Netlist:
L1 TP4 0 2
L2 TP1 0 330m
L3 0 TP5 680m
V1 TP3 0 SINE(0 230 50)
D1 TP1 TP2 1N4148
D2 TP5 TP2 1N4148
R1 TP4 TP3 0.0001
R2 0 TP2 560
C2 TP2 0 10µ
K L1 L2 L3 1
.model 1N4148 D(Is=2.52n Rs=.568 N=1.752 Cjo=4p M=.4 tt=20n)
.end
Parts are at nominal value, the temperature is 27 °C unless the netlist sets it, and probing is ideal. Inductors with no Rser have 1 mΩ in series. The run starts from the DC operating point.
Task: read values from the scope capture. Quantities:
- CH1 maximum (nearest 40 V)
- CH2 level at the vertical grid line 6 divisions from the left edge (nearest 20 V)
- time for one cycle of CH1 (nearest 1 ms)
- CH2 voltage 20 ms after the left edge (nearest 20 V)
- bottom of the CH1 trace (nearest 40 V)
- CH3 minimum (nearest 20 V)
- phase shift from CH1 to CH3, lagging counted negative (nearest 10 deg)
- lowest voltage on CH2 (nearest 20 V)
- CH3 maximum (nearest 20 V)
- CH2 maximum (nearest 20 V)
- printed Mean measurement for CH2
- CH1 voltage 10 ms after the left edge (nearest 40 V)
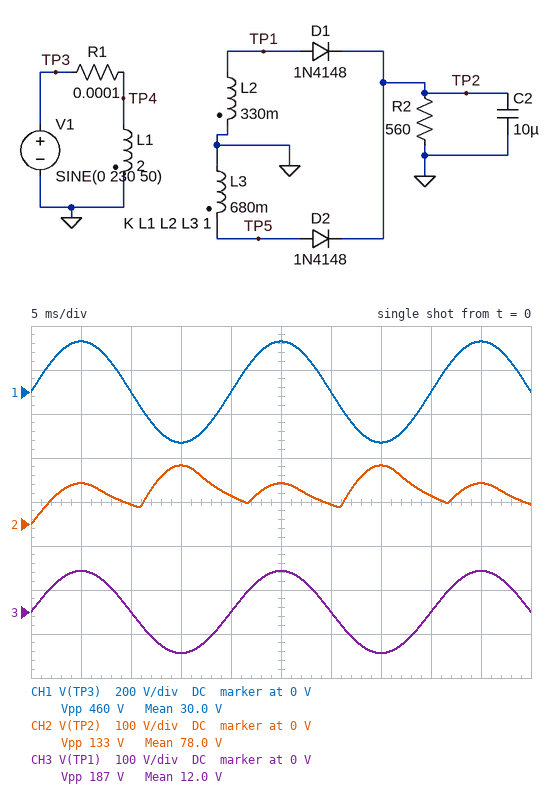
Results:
240 V
40 V
20 ms
60 V
-240 V
-100 V
0 deg
0 V
100 V
140 V
78.0 V
0 V
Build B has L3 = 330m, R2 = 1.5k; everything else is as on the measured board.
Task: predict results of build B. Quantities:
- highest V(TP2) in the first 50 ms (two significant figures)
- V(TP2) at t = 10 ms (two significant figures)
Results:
93 V
68 V
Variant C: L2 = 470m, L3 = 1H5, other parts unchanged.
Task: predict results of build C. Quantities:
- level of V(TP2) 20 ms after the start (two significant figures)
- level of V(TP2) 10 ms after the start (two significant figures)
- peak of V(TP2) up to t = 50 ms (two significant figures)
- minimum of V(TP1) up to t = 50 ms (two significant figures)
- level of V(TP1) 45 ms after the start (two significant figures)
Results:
95 V
53 V
200 V
-110 V
110 V
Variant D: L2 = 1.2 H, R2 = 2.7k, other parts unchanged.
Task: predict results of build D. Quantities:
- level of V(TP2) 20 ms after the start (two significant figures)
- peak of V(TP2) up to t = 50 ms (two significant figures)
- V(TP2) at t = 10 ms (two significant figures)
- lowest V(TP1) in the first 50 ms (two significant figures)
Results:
110 V
180 V
150 V
-180 V
